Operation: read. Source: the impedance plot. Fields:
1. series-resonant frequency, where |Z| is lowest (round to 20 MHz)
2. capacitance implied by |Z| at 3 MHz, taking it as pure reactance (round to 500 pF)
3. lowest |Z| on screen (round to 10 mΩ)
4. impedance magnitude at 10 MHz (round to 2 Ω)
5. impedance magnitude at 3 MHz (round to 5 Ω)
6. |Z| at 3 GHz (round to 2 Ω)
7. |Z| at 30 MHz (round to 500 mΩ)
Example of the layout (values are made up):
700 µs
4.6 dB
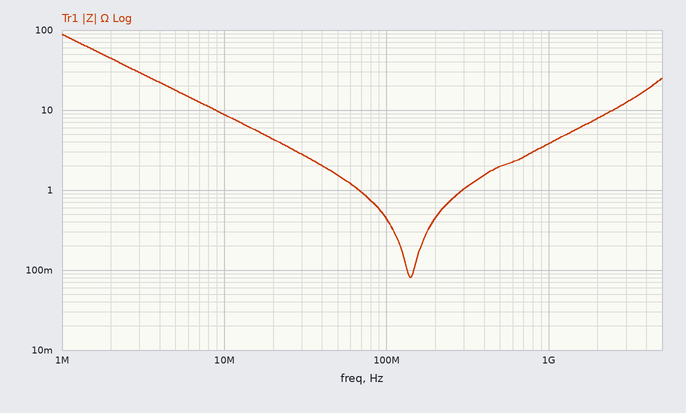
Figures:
140 MHz
2.0 nF
80 mΩ
8 Ω
30 Ω
12 Ω
3.0 Ω
